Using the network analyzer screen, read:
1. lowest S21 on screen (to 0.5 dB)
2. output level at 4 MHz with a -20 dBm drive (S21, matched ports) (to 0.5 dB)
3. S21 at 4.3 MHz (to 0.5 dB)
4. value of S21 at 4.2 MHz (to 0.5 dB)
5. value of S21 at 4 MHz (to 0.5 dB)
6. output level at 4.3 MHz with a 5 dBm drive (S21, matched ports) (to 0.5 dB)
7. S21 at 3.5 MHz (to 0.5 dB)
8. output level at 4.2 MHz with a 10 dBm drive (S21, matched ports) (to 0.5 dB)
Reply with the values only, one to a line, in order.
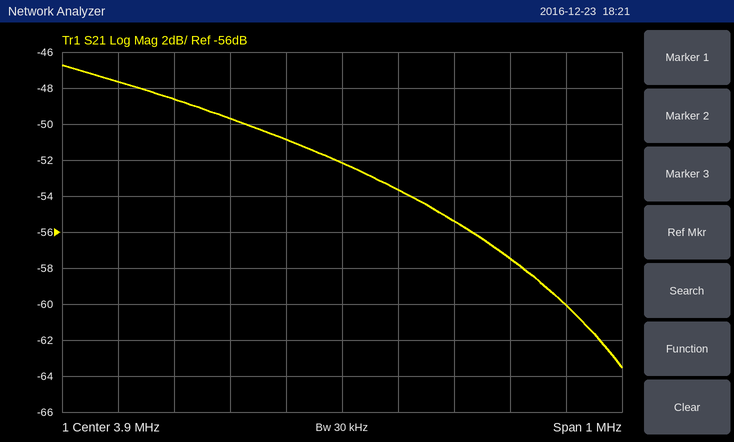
-63.5 dB
-73.5 dBm
-60.0 dB
-57.5 dB
-53.5 dB
-55.0 dBm
-47.5 dB
-47.5 dBm
